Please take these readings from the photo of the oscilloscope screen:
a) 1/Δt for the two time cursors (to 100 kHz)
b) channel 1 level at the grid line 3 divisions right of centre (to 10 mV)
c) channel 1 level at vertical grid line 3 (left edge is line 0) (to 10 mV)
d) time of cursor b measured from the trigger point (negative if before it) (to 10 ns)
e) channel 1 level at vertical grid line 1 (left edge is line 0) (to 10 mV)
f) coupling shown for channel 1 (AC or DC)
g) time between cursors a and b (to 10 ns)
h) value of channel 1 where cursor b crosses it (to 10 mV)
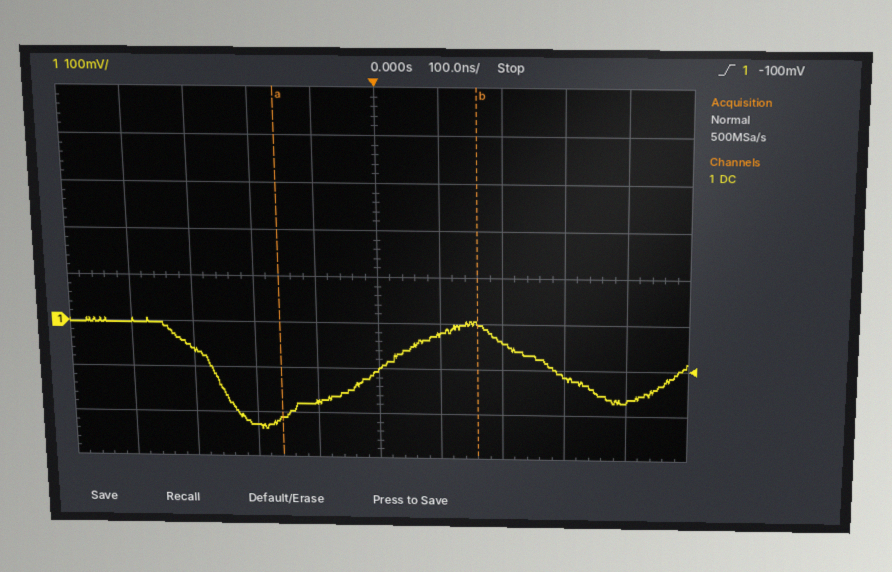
3.1 MHz
-110 mV
-230 mV
+160 ns
0 mV
DC
320 ns
0 mV
